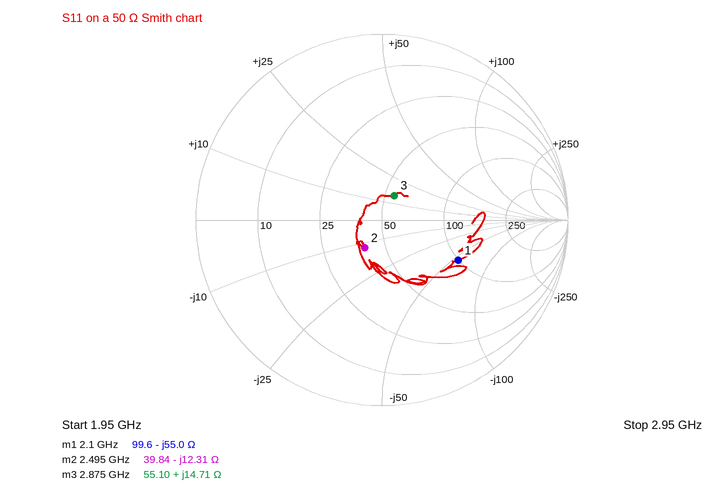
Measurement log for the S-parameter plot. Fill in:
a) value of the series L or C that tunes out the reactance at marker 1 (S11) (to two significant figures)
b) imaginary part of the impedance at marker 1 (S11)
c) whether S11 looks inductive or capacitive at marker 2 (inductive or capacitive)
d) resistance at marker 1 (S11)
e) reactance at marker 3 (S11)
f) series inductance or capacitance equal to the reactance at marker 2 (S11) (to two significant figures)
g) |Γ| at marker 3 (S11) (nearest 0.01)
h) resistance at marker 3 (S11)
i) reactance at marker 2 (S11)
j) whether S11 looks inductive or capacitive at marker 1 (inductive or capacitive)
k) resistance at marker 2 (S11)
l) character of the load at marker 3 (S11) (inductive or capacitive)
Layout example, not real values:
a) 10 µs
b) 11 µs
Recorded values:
a) 4.2 nH
b) -55.0 Ω
c) capacitive
d) 99.6 Ω
e) +14.71 Ω
f) 5.2 pF
g) 0.15
h) 55.10 Ω
i) -12.31 Ω
j) capacitive
k) 39.84 Ω
l) inductive
